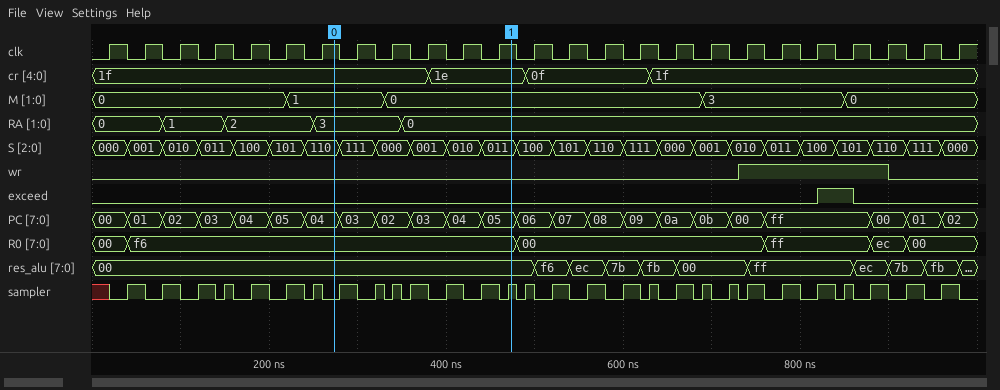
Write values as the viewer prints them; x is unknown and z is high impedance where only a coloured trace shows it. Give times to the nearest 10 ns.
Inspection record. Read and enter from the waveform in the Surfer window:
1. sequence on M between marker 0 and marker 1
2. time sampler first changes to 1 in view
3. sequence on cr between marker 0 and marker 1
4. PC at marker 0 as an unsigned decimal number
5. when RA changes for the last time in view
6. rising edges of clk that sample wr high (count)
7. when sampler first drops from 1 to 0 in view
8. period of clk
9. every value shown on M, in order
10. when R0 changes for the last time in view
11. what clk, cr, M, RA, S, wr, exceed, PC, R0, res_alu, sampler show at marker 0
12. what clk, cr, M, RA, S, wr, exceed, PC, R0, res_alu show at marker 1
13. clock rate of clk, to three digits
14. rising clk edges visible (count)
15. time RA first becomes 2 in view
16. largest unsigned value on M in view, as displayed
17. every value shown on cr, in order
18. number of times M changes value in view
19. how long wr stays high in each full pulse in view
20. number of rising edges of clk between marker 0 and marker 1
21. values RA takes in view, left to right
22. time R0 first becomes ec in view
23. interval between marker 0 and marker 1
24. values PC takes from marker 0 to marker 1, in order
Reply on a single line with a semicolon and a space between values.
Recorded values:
1, 0; 40 ns; 1f, 1e; 4; 350 ns; 5; 60 ns; 40 ns; 0, 1, 0, 3, 0; 920 ns; clk=1, cr=1f, M=1, RA=3, S=110, wr=0, exceed=0, PC=04, R0=f6, res_alu=00, sampler=0; clk=1, cr=1e, M=0, RA=0, S=011, wr=0, exceed=0, PC=05, R0=f6, res_alu=00; 25.0 MHz; 25; 150 ns; 3; 1f, 1e, 0f, 1f; 4; 170 ns; 5; 0, 1, 2, 3, 0; 880 ns; 200 ns; 04, 03, 02, 03, 04, 05
